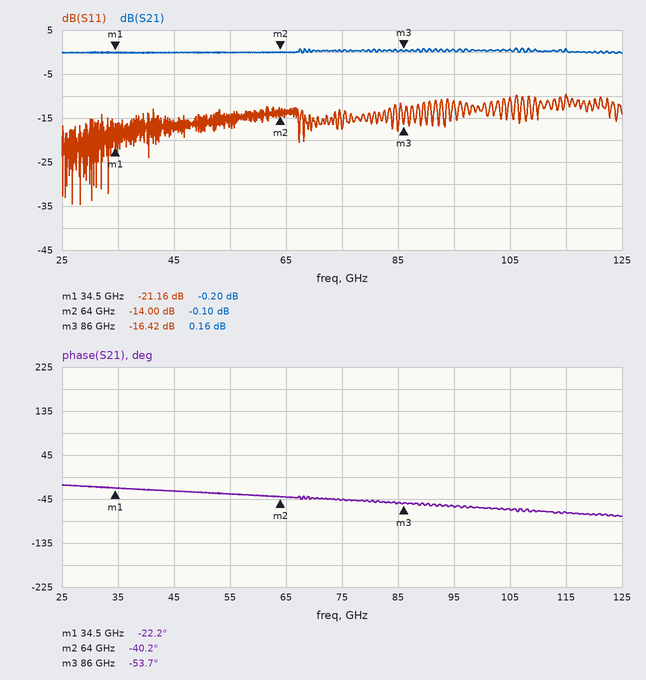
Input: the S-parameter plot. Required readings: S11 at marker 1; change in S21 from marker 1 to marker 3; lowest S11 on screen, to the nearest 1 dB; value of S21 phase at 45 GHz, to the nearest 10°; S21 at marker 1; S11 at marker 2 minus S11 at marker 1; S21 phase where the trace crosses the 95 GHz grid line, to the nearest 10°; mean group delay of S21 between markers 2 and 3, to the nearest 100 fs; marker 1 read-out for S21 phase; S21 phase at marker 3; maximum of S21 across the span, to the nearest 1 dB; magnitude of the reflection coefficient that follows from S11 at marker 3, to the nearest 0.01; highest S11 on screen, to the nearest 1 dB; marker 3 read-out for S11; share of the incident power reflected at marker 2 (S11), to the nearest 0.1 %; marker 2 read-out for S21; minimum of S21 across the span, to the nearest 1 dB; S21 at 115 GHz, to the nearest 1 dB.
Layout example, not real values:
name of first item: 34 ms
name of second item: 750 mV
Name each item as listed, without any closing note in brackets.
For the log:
S11 at marker 1: -21.16 dB
change in S21 from marker 1 to marker 3: 0.36 dB
lowest S11 on screen, to the nearest 1 dB: -35 dB
value of S21 phase at 45 GHz, to the nearest 10°: -30°
S21 at marker 1: -0.20 dB
S11 at marker 2 minus S11 at marker 1: 7.16 dB
S21 phase where the trace crosses the 95 GHz grid line, to the nearest 10°: -60°
mean group delay of S21 between markers 2 and 3, to the nearest 100 fs: 1.7 ps
marker 1 read-out for S21 phase: -22.2°
S21 phase at marker 3: -53.7°
maximum of S21 across the span, to the nearest 1 dB: 1 dB
magnitude of the reflection coefficient that follows from S11 at marker 3, to the nearest 0.01: 0.15
highest S11 on screen, to the nearest 1 dB: -10 dB
marker 3 read-out for S11: -16.42 dB
share of the incident power reflected at marker 2 (S11), to the nearest 0.1 %: 4.0 %
marker 2 read-out for S21: -0.10 dB
minimum of S21 across the span, to the nearest 1 dB: 0 dB
S21 at 115 GHz, to the nearest 1 dB: 1 dB
